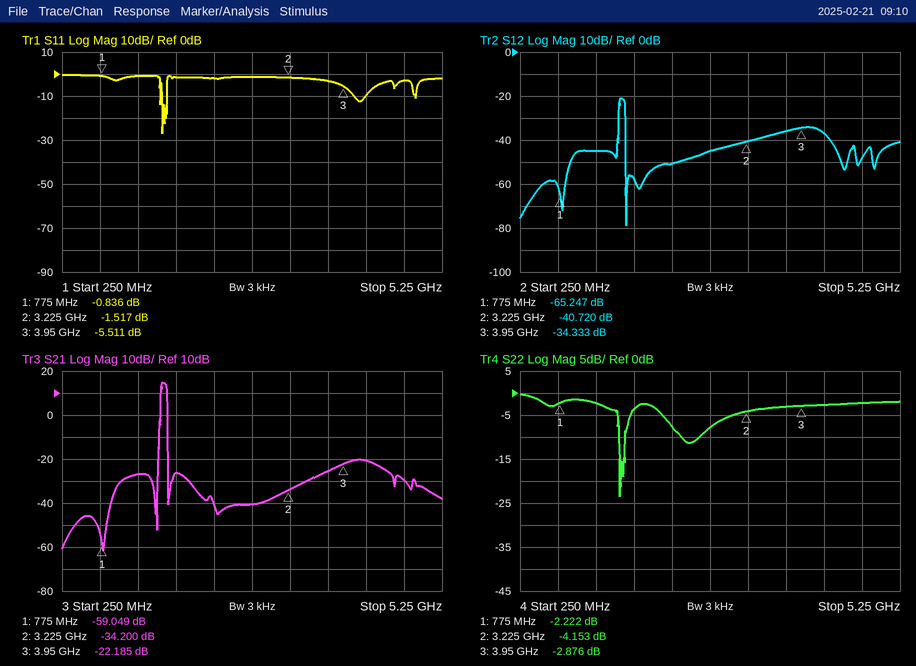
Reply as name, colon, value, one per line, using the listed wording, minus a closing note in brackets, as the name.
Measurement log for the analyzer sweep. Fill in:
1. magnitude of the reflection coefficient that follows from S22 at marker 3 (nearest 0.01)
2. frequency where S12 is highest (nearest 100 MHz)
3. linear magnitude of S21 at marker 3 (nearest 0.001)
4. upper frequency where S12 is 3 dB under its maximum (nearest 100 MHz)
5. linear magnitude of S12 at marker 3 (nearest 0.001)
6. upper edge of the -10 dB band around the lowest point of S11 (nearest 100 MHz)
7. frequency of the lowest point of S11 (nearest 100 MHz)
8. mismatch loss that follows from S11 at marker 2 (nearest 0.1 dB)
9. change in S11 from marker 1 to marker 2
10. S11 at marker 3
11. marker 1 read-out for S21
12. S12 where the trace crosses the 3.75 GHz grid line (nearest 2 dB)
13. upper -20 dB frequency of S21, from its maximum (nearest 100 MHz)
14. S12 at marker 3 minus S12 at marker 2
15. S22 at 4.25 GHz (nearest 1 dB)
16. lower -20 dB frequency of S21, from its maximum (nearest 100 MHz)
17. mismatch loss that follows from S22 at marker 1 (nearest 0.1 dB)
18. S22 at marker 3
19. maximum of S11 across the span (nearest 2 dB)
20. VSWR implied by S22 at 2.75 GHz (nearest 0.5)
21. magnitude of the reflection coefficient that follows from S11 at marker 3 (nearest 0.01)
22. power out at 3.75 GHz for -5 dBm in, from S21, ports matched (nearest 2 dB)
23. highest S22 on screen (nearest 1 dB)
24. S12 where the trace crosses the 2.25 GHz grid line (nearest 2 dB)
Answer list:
magnitude of the reflection coefficient that follows from S22 at marker 3: 0.72
frequency where S12 is highest: 1.6 GHz
linear magnitude of S21 at marker 3: 0.078
upper frequency where S12 is 3 dB under its maximum: 1.6 GHz
linear magnitude of S12 at marker 3: 0.019
upper edge of the -10 dB band around the lowest point of S11: 1.6 GHz
frequency of the lowest point of S11: 1.6 GHz
mismatch loss that follows from S11 at marker 2: 5.3 dB
change in S11 from marker 1 to marker 2: -0.681 dB
S11 at marker 3: -5.511 dB
marker 1 read-out for S21: -59.049 dB
S12 where the trace crosses the 3.75 GHz grid line: -36 dB
upper -20 dB frequency of S21, from its maximum: 1.6 GHz
S12 at marker 3 minus S12 at marker 2: 6.387 dB
S22 at 4.25 GHz: -3 dB
lower -20 dB frequency of S21, from its maximum: 1.5 GHz
mismatch loss that follows from S22 at marker 1: 4.0 dB
S22 at marker 3: -2.876 dB
maximum of S11 across the span: 0 dB
VSWR implied by S22 at 2.75 GHz: 2.5
magnitude of the reflection coefficient that follows from S11 at marker 3: 0.53
power out at 3.75 GHz for -5 dBm in, from S21, ports matched: -30 dBm
highest S22 on screen: 0 dB
S12 where the trace crosses the 2.25 GHz grid line: -50 dB
